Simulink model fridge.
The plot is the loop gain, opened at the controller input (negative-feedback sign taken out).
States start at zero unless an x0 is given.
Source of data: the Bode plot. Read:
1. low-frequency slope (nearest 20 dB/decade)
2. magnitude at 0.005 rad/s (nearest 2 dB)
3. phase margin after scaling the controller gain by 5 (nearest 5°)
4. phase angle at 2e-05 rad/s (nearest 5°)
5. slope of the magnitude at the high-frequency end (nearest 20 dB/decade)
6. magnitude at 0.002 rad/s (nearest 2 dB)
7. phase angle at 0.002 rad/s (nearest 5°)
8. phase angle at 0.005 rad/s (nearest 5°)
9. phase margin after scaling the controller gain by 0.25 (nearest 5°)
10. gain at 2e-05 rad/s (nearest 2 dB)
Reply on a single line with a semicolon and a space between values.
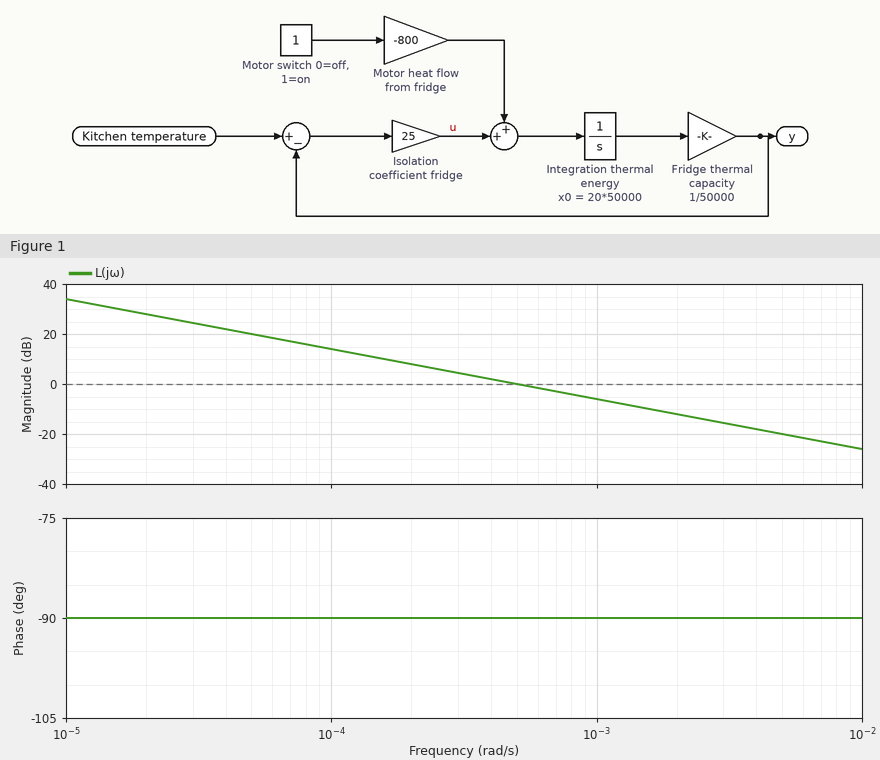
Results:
-20 dB/decade; -20 dB; 90°; -90°; -20 dB/decade; -12 dB; -90°; -90°; 90°; 28 dB
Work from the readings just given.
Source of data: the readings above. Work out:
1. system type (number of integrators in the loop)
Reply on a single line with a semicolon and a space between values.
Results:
1
